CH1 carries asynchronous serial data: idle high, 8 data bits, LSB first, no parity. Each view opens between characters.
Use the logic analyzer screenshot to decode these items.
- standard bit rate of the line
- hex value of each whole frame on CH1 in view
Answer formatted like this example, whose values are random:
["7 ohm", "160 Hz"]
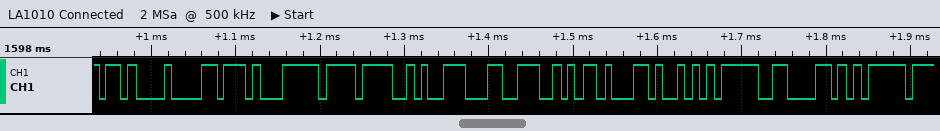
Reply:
["115200 baud", "0B, D8, F1, EF, CA, CC, 6A, 2C, F5, 86, F5"]
